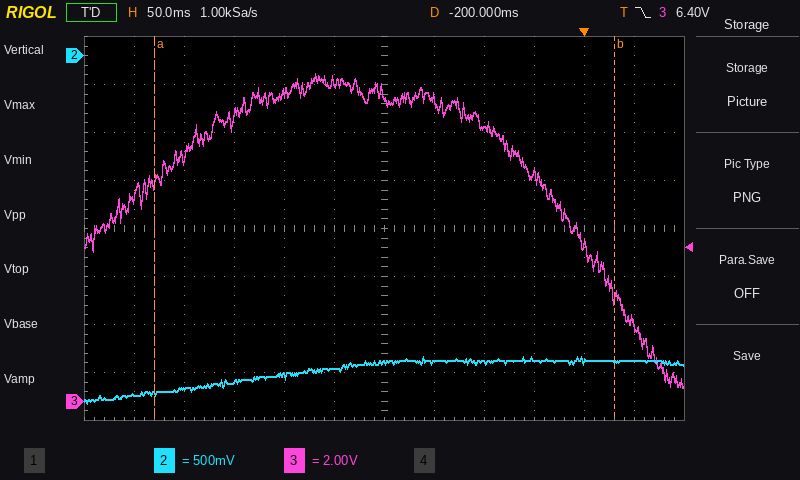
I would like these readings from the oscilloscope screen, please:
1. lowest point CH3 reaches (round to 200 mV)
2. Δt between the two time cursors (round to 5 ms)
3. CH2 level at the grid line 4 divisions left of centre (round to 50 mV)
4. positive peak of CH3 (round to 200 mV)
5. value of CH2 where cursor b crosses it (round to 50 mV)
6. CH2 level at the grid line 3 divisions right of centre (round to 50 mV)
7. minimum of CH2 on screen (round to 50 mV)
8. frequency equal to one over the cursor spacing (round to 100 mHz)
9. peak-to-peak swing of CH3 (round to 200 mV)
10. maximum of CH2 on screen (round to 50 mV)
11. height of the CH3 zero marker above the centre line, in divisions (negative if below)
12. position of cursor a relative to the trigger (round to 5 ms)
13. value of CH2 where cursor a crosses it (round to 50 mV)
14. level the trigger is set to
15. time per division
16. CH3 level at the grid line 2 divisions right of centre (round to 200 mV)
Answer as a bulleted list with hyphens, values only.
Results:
- 600 mV
- 460 ms
- -3.45 V
- 13.6 V
- -3.20 V
- -3.15 V
- -3.60 V
- 2.2 Hz
- 13.0 V
- -3.15 V
- -3.6 div
- -430 ms
- -3.50 V
- 6.40 V
- 50 ms
- 11.4 V
